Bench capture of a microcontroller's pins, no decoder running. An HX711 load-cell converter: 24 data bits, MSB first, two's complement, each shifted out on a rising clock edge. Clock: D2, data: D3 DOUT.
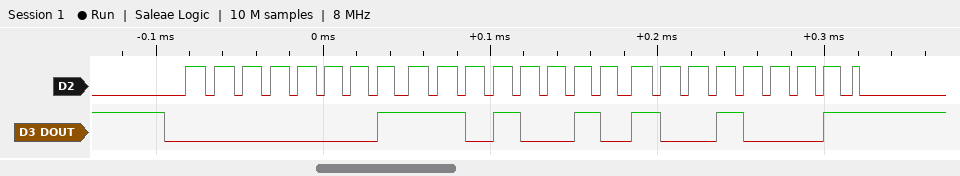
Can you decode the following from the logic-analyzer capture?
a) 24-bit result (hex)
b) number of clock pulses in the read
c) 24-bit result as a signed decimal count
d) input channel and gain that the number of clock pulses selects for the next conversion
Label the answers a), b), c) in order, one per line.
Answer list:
a) 0x01D291
b) 25
c) 119441
d) channel A, gain 128
